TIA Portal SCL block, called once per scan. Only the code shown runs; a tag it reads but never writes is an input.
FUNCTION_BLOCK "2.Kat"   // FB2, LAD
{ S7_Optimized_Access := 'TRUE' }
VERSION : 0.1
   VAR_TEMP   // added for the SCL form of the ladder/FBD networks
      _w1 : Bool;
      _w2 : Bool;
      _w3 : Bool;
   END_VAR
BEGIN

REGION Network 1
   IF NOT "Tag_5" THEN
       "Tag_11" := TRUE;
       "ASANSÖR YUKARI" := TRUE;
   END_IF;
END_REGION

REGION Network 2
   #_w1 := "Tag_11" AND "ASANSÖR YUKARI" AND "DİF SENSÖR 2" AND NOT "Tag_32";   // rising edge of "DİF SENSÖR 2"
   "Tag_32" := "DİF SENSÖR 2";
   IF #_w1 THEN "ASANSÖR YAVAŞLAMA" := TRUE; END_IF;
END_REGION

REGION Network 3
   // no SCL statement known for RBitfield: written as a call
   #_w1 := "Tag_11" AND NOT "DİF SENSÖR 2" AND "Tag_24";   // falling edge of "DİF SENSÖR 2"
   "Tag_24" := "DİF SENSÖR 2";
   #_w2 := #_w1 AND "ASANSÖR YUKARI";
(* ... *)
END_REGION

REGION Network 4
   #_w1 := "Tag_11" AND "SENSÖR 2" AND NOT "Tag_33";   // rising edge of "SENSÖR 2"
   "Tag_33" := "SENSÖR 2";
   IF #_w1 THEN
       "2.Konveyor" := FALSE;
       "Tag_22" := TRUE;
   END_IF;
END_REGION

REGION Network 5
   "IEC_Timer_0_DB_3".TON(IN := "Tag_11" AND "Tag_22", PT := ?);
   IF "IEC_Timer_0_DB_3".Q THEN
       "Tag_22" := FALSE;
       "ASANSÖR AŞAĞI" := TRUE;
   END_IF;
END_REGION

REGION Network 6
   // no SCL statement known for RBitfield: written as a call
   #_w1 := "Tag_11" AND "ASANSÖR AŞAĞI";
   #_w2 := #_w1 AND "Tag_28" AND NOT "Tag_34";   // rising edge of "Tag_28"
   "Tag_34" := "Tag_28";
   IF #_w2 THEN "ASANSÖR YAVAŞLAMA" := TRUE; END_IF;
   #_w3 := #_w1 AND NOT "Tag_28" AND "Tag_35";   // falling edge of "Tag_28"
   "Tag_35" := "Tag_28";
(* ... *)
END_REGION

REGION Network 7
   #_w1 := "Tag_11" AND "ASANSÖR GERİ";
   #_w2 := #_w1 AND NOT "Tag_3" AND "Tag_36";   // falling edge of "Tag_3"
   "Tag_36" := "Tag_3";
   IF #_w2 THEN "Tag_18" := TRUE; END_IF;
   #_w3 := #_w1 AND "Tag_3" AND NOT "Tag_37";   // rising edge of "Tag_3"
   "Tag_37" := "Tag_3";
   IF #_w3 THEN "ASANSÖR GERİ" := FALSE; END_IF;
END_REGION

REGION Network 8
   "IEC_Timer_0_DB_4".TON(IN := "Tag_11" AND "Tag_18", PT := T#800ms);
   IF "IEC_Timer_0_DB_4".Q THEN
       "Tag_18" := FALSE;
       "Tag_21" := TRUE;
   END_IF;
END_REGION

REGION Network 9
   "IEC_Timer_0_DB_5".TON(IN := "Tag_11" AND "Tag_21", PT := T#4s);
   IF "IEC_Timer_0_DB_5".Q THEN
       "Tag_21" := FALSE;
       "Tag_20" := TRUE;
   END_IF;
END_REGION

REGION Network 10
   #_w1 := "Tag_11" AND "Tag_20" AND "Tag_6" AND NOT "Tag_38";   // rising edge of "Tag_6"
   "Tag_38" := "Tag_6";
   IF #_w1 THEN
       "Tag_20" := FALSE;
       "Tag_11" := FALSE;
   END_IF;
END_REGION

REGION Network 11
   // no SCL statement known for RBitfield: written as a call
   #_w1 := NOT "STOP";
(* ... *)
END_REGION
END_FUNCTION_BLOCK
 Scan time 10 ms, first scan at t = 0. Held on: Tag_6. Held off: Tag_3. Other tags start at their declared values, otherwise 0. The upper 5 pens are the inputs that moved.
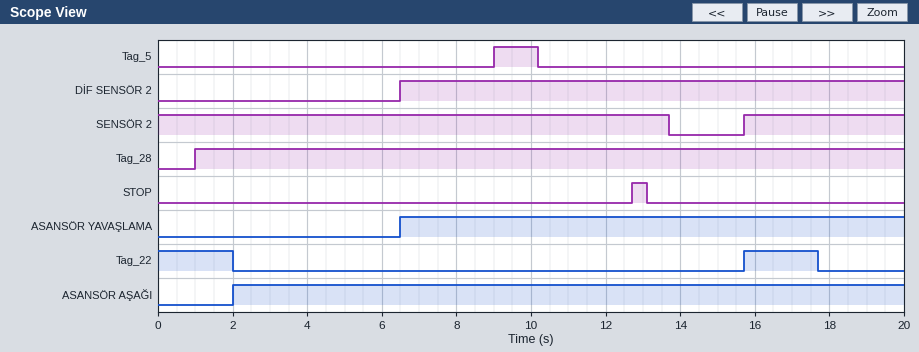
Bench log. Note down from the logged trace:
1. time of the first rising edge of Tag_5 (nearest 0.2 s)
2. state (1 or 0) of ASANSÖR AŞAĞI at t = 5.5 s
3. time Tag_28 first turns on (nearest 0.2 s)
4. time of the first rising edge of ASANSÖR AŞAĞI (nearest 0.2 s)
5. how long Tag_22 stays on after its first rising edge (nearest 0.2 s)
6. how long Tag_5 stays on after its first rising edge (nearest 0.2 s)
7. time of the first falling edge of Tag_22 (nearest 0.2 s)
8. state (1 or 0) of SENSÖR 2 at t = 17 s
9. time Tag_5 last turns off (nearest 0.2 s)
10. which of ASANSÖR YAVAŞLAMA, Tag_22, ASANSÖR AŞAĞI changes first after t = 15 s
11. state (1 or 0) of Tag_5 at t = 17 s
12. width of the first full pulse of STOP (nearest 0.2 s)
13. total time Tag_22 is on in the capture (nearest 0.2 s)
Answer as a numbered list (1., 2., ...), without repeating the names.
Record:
1. 9.0 s
2. 1
3. 1.0 s
4. 2.0 s
5. 2.0 s
6. 1.2 s
7. 2.0 s
8. 1
9. 10.2 s
10. Tag_22
11. 0
12. 0.4 s
13. 4.0 s
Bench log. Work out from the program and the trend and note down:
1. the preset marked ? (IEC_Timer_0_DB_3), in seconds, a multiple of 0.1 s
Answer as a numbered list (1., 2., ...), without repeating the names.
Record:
1. 2.0 s
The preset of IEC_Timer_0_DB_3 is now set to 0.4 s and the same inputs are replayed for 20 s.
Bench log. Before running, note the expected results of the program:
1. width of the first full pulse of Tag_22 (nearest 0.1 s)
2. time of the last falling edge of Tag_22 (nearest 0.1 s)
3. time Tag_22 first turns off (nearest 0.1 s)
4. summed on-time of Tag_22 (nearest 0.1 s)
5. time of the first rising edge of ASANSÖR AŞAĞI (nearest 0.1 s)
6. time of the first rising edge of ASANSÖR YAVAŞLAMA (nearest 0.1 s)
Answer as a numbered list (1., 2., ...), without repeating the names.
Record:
1. 0.4 s
2. 16.1 s
3. 0.4 s
4. 0.8 s
5. 0.4 s
6. 1.0 s
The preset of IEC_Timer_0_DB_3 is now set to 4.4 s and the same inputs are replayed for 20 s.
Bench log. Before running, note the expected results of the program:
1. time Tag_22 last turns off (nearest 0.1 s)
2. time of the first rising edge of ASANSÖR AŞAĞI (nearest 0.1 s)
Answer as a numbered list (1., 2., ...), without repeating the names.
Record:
1. 4.4 s
2. 4.4 s
